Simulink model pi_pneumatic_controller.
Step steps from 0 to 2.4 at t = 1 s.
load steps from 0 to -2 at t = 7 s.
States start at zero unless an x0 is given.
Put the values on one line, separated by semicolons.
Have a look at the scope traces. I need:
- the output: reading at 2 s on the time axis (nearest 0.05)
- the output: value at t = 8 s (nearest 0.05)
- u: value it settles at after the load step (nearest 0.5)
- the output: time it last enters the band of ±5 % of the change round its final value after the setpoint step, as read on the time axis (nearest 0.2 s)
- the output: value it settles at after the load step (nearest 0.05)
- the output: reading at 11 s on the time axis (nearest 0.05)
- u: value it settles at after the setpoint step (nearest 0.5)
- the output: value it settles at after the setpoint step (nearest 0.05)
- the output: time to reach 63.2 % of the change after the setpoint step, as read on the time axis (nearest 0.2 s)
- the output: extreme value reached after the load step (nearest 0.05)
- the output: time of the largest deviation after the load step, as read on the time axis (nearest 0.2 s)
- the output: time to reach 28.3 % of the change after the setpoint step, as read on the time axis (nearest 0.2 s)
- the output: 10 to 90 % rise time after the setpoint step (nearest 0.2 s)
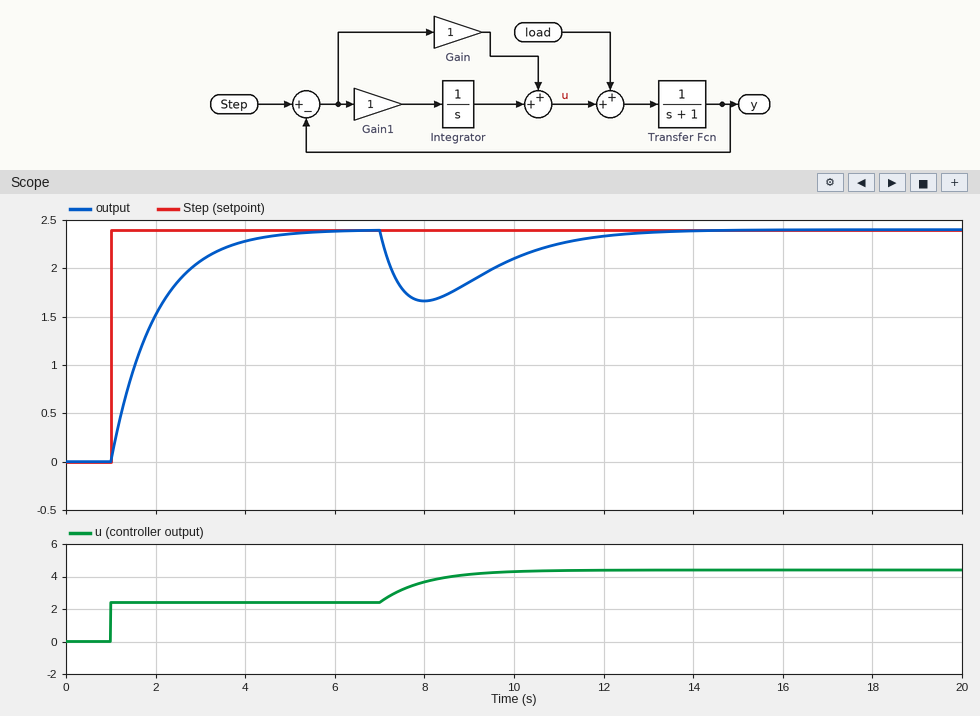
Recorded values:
1.50; 1.65; 4.5; 4.0 s; 2.40; 2.25; 2.5; 2.40; 2.0 s; 1.65; 8.0 s; 1.4 s; 2.2 s
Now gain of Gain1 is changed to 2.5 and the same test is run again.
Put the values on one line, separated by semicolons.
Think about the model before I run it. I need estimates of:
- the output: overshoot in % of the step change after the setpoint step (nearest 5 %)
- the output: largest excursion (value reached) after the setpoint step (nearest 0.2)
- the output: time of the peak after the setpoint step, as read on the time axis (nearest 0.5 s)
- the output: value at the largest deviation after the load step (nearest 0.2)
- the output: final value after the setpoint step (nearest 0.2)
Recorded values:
10 %; 2.6; 3.0 s; 1.8; 2.4
